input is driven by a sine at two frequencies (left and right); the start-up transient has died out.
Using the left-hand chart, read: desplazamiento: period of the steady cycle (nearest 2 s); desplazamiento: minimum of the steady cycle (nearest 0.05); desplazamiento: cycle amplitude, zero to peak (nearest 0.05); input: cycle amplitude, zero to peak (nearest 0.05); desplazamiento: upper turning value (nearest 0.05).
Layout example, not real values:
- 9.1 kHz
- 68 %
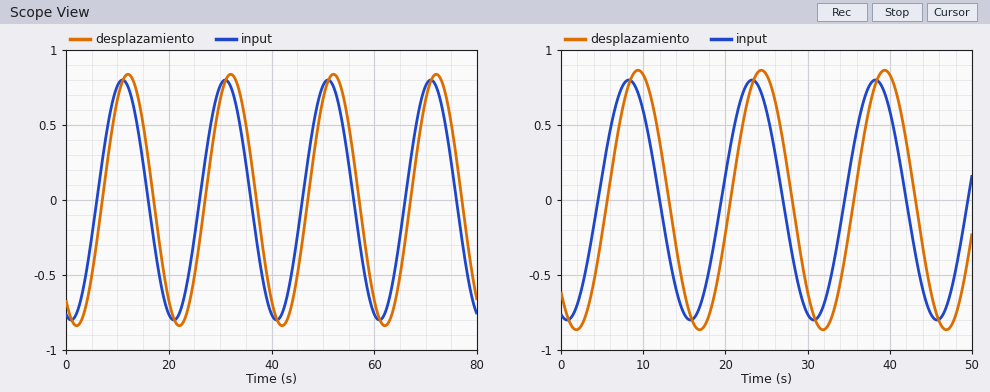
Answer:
- 20 s
- -0.85
- 0.85
- 0.80
- 0.85
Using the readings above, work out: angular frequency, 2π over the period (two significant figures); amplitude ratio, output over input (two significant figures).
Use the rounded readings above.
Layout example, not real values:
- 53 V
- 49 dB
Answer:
- 0.31 rad/s
- 1.1
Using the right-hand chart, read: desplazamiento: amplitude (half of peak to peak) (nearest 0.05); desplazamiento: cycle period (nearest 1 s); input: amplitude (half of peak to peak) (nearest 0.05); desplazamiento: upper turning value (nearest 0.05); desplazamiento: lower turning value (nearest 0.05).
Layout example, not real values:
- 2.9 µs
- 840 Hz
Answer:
- 0.85
- 15 s
- 0.80
- 0.85
- -0.85
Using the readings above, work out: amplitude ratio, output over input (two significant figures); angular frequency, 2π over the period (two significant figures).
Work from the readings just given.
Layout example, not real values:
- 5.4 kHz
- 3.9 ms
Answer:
- 1.1
- 0.42 rad/s
